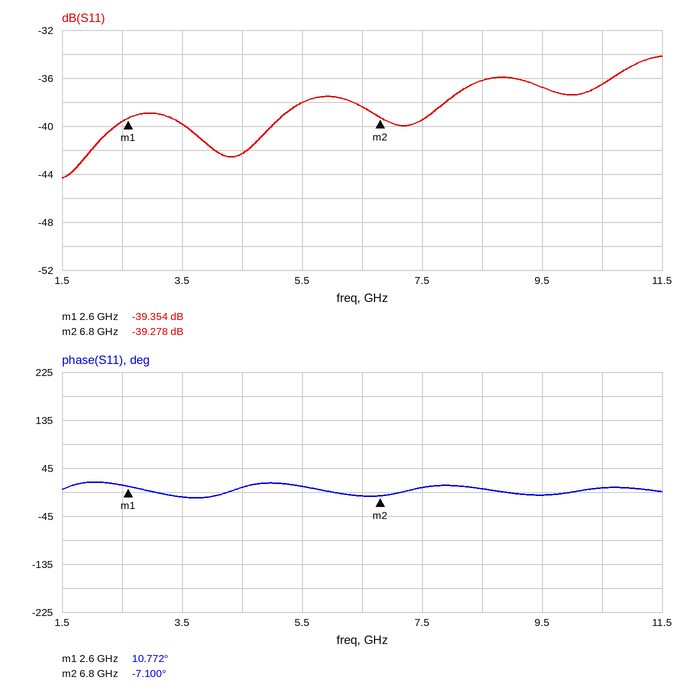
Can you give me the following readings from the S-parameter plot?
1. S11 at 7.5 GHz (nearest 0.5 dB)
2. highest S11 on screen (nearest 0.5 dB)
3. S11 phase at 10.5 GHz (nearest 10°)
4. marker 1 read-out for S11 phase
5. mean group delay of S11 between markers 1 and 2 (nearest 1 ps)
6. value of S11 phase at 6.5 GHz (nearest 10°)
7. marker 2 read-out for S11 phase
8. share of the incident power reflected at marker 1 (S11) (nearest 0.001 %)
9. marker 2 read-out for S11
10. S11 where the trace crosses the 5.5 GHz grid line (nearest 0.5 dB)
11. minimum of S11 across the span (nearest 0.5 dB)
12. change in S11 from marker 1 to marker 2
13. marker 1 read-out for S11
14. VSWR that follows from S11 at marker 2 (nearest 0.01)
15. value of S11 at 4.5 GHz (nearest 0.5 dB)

-39.5 dB
-34.0 dB
10°
10.772°
12 ps
-10°
-7.100°
0.012 %
-39.278 dB
-38.0 dB
-44.5 dB
0.076 dB
-39.354 dB
1.02
-42.5 dB
